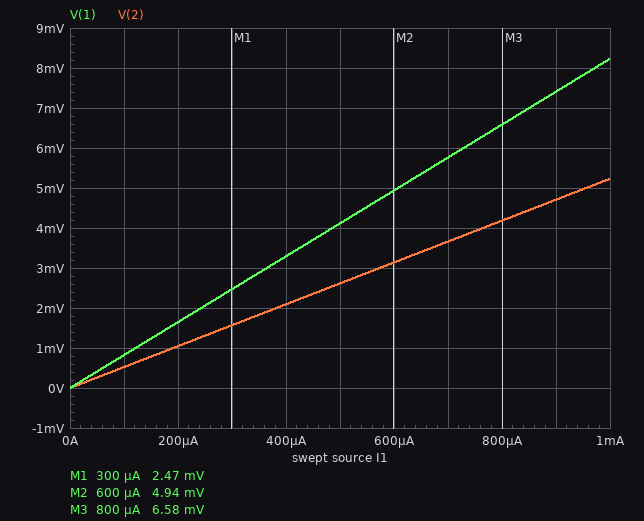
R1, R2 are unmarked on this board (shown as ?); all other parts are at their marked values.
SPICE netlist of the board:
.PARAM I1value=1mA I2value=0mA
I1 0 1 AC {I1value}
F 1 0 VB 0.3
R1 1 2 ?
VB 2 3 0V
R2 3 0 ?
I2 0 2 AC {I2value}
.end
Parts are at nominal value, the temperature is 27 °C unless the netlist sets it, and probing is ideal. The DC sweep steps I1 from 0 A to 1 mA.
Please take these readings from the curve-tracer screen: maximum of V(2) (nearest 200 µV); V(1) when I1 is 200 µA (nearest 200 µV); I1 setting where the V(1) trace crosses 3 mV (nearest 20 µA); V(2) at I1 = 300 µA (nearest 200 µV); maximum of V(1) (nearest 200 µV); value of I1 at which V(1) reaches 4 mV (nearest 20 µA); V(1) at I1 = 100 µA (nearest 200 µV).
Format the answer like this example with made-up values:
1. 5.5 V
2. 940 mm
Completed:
1. 5.2 mV
2. 1.6 mV
3. 360 µA
4. 1.6 mV
5. 8.2 mV
6. 480 µA
7. 800 µV
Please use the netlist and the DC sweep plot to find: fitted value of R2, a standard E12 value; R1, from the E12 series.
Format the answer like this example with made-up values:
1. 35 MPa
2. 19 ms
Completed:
1. 6.8 Ω
2. 3.9 Ω
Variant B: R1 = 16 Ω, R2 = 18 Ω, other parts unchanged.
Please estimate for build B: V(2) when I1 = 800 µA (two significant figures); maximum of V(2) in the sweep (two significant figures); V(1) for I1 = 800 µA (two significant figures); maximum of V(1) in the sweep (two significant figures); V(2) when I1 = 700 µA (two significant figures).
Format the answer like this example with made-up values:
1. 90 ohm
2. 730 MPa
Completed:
1. 11 mV
2. 14 mV
3. 21 mV
4. 26 mV
5. 9.7 mV
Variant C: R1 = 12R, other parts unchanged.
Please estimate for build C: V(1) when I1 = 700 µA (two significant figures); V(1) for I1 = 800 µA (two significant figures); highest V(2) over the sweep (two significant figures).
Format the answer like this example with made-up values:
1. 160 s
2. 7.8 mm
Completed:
1. 10 mV
2. 12 mV
3. 5.2 mV
